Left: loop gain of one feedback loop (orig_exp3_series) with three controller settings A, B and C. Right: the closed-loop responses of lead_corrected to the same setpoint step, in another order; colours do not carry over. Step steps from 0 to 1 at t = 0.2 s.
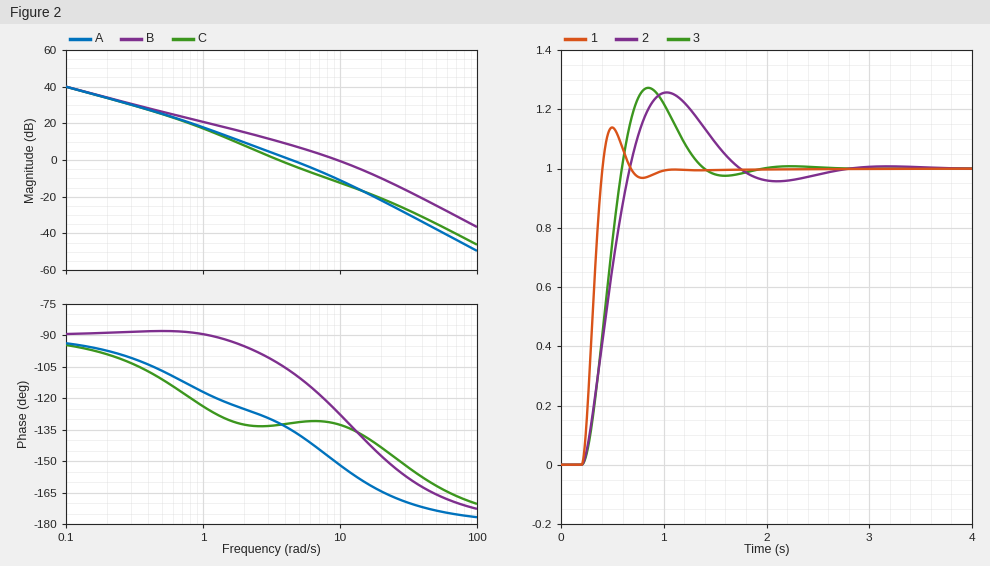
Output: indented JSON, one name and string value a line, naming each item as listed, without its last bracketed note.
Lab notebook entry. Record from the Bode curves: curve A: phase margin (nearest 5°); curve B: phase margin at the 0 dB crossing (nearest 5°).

{
  "curve A: phase margin": "45°",
  "curve B: phase margin at the 0 dB crossing": "55°"
}
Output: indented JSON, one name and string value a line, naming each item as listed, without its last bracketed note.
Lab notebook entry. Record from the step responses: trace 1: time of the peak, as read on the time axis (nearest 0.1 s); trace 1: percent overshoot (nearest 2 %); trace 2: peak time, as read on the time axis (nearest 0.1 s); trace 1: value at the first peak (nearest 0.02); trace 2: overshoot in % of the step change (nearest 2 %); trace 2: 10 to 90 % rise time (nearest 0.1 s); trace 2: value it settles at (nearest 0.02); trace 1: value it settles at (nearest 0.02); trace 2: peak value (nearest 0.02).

{
  "trace 1: time of the peak, as read on the time axis": "0.5 s",
  "trace 1: percent overshoot": "14 %",
  "trace 2: peak time, as read on the time axis": "1.0 s",
  "trace 1: value at the first peak": "1.14",
  "trace 2: overshoot in % of the step change": "26 %",
  "trace 2: 10 to 90 % rise time": "0.3 s",
  "trace 2: value it settles at": "1.00",
  "trace 1: value it settles at": "1.00",
  "trace 2: peak value": "1.26"
}
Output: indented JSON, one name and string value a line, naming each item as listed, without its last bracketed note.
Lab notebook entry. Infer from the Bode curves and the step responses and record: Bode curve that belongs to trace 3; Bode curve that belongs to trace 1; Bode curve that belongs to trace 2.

{
  "Bode curve that belongs to trace 3": "A",
  "Bode curve that belongs to trace 1": "B",
  "Bode curve that belongs to trace 2": "C"
}
